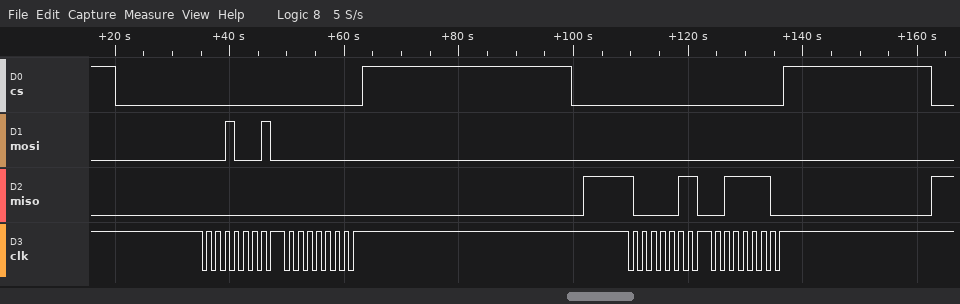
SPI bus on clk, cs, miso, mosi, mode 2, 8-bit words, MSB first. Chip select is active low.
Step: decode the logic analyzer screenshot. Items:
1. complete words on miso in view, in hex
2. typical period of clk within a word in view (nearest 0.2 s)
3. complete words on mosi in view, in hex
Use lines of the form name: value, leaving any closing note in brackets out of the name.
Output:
complete words on miso in view, in hex: 00, 00, 83, 3E
typical period of clk within a word in view: 1.6 s
complete words on mosi in view, in hex: 11, 00, 00, 00
